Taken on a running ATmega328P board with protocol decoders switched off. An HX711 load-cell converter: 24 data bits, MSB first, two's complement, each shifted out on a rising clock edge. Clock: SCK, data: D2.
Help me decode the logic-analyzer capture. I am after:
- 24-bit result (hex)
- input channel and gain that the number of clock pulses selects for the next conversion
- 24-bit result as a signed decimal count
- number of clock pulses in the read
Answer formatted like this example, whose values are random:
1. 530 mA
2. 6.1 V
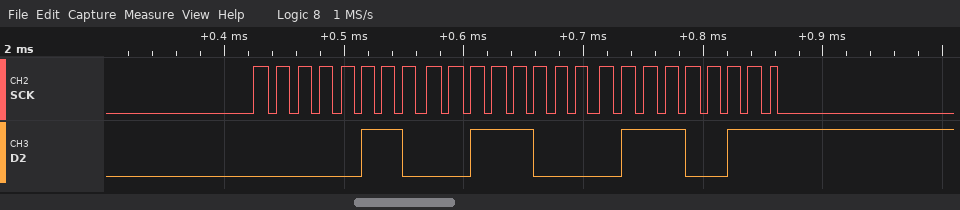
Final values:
1. 0x063873
2. channel A, gain 128
3. 407667
4. 25
